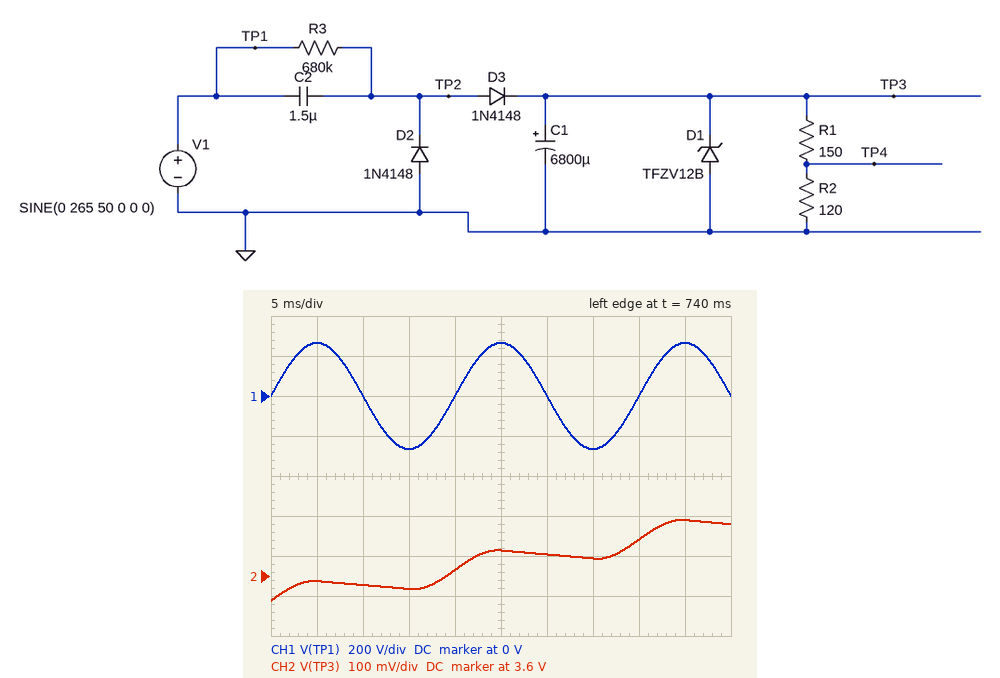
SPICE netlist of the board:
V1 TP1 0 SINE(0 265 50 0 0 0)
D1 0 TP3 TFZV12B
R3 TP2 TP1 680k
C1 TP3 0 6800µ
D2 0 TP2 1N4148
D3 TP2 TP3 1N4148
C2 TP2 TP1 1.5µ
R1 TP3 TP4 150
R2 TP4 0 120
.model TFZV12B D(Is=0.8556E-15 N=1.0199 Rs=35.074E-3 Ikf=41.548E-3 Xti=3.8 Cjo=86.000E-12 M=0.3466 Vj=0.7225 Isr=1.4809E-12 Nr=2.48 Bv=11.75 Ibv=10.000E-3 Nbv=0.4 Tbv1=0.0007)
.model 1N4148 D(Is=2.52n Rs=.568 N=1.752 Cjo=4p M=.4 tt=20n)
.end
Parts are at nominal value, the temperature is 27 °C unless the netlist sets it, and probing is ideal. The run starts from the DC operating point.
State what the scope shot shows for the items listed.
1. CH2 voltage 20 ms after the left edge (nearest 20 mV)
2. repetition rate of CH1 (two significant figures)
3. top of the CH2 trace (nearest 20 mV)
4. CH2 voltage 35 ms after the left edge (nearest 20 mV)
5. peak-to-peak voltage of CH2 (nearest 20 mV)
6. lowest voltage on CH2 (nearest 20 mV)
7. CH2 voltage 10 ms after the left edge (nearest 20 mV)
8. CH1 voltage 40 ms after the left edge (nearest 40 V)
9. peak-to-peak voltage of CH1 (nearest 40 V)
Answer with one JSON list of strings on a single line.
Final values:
["3.62 V", "50 Hz", "3.74 V", "3.64 V", "200 mV", "3.54 V", "3.58 V", "0 V", "520 V"]
